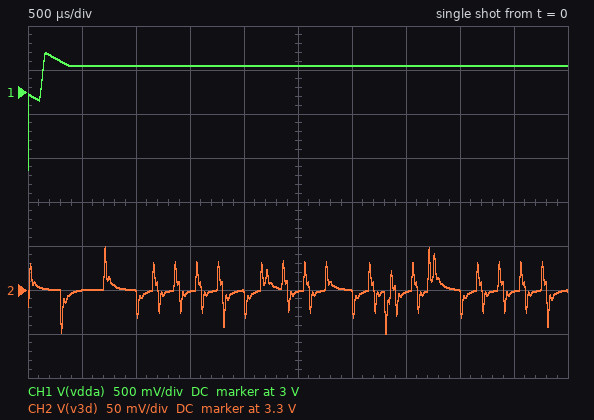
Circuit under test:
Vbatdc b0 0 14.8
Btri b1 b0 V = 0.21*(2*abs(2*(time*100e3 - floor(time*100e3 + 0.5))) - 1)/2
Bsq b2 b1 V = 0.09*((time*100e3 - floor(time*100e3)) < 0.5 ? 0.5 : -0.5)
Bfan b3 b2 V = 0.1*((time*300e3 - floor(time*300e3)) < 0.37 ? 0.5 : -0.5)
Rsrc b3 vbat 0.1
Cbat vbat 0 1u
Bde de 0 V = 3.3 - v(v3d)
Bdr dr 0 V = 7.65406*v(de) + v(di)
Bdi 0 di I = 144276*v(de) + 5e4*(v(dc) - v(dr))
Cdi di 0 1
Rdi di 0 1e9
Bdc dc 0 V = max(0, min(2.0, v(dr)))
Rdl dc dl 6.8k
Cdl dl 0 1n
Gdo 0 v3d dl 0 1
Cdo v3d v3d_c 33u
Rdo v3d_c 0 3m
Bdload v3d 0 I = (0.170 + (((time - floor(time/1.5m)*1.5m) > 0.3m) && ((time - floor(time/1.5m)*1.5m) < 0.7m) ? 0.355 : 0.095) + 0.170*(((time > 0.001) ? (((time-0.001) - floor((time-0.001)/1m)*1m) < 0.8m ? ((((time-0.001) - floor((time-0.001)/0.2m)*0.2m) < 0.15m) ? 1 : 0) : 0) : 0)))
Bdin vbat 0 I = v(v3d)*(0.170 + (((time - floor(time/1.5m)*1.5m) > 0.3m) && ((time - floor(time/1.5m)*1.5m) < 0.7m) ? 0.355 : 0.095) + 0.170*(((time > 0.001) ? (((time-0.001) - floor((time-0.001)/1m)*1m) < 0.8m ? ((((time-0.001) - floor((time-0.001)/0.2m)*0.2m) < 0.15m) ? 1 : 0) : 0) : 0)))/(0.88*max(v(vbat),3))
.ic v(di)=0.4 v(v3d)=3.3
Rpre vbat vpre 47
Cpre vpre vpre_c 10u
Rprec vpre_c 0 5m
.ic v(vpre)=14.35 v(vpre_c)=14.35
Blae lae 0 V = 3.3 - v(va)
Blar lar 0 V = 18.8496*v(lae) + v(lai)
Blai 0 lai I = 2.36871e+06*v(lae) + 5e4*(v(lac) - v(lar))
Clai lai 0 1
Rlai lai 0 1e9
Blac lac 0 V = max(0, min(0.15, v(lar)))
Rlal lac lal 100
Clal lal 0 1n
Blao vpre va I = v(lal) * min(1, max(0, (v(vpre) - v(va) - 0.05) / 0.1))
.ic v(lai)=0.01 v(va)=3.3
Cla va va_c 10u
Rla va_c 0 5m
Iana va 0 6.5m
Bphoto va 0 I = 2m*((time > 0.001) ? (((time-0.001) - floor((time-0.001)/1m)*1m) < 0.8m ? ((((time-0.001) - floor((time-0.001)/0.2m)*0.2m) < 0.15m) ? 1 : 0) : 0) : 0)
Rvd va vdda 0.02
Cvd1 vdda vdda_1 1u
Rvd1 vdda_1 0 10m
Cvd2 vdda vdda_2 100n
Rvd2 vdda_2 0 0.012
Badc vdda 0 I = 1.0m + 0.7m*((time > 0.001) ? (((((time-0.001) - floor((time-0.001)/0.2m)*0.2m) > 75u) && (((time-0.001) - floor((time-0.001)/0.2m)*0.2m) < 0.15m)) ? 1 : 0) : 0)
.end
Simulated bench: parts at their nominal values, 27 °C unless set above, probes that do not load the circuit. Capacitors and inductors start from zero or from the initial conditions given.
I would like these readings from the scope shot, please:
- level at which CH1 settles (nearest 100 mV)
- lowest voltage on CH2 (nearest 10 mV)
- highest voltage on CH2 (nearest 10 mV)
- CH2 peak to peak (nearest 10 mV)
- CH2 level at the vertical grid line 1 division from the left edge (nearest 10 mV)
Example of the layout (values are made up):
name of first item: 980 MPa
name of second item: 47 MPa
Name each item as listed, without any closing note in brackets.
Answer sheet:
level at which CH1 settles: 3.3 V
lowest voltage on CH2: 3.25 V
highest voltage on CH2: 3.35 V
CH2 peak to peak: 100 mV
CH2 level at the vertical grid line 1 division from the left edge: 3.30 V
